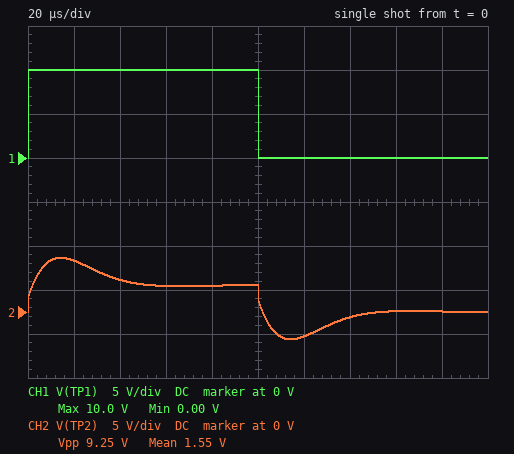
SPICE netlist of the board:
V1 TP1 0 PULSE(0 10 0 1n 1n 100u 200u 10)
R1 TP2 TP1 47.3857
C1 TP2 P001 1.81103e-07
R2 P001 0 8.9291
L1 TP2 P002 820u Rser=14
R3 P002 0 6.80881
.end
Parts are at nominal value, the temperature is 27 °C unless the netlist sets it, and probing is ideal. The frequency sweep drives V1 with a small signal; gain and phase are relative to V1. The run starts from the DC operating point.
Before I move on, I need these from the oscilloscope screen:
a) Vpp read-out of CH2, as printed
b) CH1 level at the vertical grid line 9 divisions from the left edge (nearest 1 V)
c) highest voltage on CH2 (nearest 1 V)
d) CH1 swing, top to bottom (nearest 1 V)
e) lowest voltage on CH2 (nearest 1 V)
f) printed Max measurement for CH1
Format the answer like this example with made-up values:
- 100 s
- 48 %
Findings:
- 9.25 V
- 0 V
- 6 V
- 10 V
- -3 V
- 10.0 V
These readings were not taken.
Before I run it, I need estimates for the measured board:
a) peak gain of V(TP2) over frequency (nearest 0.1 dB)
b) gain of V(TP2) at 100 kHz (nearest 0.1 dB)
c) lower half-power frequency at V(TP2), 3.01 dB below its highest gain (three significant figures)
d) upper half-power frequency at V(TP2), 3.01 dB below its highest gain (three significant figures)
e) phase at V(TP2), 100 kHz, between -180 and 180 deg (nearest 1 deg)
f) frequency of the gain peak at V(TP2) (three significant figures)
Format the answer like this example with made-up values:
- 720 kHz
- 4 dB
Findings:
- -2.2 dB
- -13.1 dB
- 6.32 kHz
- 28.4 kHz
- -35 deg
- 13.9 kHz
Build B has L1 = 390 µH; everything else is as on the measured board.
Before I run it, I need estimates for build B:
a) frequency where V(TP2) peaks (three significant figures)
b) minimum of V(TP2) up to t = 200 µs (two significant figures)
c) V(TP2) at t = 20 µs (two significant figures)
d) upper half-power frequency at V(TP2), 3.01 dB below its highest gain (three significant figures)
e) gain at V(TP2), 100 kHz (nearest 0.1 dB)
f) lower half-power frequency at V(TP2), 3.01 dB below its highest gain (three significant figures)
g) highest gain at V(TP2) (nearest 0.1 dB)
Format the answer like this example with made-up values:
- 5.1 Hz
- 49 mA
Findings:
- 19.8 kHz
- -2.1 V
- 4.3 V
- 38.2 kHz
- -13.0 dB
- 8.93 kHz
- -3.9 dB
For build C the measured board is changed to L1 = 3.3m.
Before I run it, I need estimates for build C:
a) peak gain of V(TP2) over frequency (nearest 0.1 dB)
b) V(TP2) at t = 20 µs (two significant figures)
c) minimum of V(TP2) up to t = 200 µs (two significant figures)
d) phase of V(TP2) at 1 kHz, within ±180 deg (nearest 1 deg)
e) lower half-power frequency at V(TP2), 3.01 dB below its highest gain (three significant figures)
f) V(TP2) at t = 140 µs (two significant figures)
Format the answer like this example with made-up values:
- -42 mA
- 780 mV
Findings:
- -0.6 dB
- 7.9 V
- -4.3 V
- 27 deg
- 2.36 kHz
- -3.7 V
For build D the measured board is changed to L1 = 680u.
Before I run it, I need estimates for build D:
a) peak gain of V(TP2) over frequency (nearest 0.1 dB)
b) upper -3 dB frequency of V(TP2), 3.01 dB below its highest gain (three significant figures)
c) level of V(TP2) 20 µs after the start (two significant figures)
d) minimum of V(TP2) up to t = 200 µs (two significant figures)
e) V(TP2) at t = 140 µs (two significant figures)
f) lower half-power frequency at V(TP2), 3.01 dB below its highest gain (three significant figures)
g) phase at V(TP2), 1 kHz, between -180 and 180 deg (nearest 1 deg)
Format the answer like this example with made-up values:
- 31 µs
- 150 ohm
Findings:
- -2.6 dB
- 30.4 kHz
- 5.4 V
- -2.8 V
- -280 mV
- 7.01 kHz
- 7 deg
